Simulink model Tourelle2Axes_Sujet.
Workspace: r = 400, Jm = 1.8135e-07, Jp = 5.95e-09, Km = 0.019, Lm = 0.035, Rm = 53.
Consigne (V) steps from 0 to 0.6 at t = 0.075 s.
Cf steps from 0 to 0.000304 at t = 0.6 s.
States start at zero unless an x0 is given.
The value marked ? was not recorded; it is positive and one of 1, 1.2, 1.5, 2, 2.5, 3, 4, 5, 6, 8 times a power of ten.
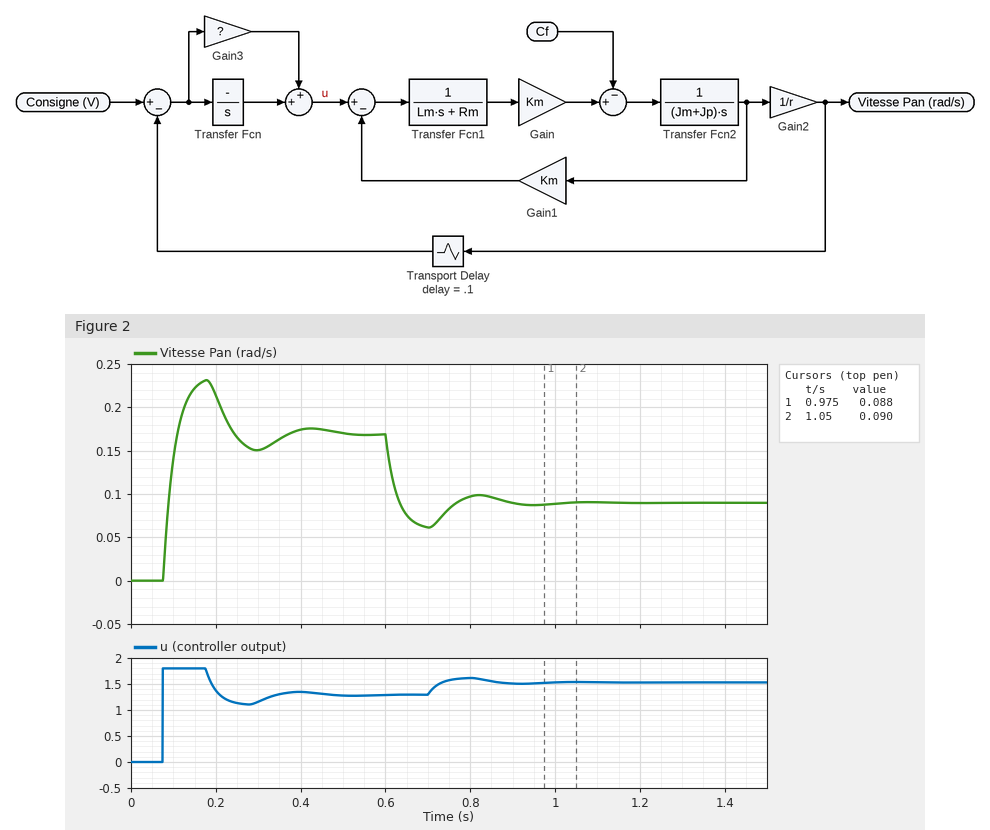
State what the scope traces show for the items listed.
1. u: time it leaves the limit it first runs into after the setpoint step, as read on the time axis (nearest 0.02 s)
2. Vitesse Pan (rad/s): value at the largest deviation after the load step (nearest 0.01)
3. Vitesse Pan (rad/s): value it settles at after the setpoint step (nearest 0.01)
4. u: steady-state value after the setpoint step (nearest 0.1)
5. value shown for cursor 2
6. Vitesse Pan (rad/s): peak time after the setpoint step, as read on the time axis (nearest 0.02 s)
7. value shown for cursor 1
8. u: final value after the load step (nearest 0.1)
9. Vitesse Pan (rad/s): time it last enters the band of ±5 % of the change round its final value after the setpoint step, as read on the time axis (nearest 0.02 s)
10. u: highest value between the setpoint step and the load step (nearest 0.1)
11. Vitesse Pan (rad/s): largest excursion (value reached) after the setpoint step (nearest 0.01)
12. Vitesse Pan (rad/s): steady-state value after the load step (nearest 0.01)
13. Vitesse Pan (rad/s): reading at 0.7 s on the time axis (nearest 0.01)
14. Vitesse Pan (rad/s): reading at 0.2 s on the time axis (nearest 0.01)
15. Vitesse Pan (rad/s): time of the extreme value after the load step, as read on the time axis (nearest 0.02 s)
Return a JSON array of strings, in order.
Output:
["0.18 s", "0.06", "0.17", "1.3", "0.090", "0.18 s", "0.088", "1.5", "0.34 s", "1.8", "0.23", "0.09", "0.06", "0.21", "0.70 s"]
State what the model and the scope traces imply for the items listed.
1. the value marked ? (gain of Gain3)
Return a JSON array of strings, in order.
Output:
["3"]
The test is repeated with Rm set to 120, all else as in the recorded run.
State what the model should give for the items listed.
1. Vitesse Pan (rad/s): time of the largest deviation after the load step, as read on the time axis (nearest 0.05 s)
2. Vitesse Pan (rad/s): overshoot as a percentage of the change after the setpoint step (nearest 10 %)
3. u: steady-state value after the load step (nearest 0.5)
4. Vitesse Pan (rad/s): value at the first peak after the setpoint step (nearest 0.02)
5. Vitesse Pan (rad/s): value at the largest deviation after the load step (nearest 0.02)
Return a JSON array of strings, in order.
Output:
["0.75 s", "20 %", "2.0", "0.20", "-0.04"]
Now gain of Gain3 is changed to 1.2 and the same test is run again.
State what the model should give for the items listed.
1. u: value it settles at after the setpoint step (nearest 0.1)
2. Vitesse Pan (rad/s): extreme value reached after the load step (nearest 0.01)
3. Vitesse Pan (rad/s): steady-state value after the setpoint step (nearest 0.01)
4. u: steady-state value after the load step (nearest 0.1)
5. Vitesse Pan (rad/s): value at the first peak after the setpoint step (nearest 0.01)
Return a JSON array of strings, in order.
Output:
["0.6", "-0.03", "0.08", "0.7", "0.09"]
